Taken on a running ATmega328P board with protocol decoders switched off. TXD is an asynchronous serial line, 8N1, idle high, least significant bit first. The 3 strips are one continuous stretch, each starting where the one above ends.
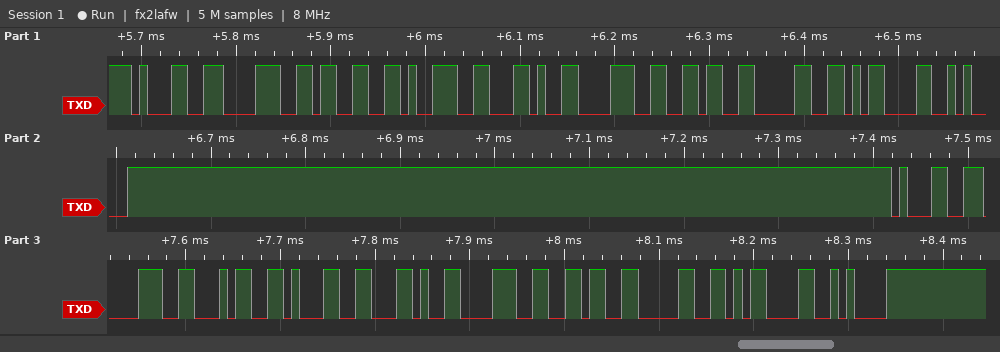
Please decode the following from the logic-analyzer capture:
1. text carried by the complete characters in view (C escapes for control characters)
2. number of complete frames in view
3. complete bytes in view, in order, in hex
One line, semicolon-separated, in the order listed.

"1839,860\r\n1841,860\r\n"; 20; 31 38 33 39 2C 38 36 30 0D 0A 31 38 34 31 2C 38 36 30 0D 0A
